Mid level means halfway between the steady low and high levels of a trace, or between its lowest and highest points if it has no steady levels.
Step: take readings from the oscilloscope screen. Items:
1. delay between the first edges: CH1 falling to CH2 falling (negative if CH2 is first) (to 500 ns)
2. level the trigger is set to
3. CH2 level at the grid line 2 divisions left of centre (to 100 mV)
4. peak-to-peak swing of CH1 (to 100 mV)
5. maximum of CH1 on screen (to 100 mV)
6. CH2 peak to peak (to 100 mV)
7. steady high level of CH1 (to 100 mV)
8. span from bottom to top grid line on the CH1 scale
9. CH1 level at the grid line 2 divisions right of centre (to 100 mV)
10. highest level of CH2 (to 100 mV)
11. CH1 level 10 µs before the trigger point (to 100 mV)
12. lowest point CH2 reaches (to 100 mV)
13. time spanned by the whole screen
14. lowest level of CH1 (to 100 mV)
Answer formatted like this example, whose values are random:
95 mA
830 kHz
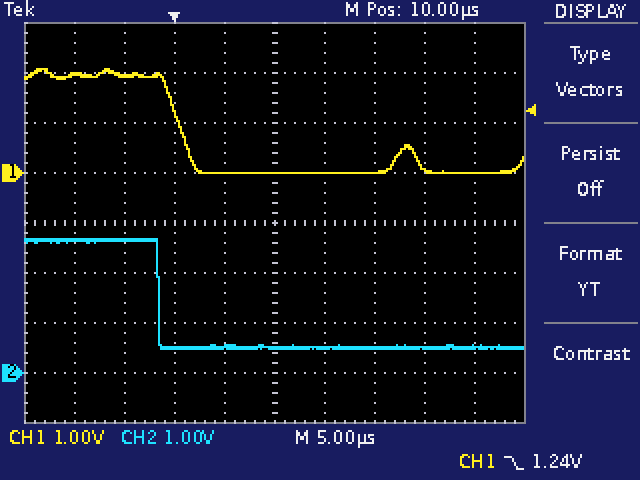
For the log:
-2.0 µs
1.24 V
500 mV
2.1 V
2.1 V
2.2 V
1.9 V
8 V
0.0 V
2.7 V
2.0 V
500 mV
50 µs
0.0 V
